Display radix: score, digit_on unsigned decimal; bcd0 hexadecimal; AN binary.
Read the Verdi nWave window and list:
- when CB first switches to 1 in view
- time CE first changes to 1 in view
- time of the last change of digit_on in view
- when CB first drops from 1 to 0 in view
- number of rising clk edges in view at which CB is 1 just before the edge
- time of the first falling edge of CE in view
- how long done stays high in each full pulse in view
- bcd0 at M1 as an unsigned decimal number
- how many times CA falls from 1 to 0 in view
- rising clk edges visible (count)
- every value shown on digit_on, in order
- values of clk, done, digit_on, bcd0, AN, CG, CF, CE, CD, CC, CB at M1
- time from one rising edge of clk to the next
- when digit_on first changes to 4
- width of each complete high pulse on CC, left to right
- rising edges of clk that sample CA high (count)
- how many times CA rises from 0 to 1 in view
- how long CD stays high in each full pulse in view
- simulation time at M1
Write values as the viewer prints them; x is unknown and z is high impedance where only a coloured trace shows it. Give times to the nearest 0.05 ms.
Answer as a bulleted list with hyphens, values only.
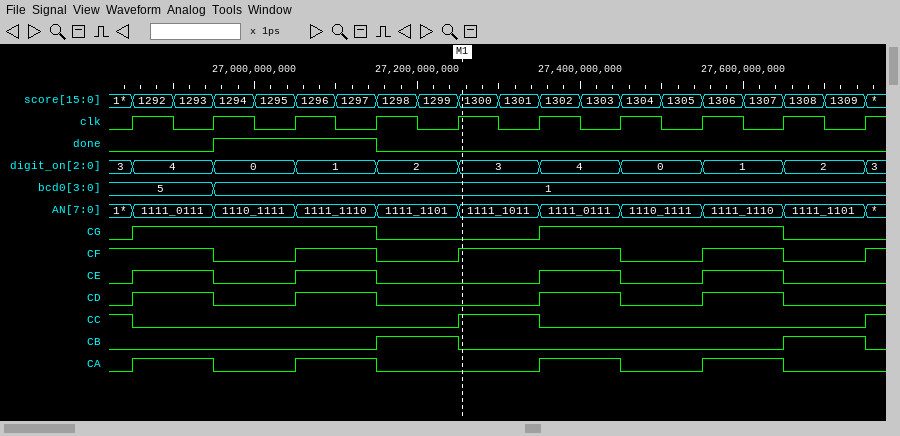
- 27.15 ms
- 26.85 ms
- 27.75 ms
- 27.25 ms
- 2
- 26.95 ms
- 0.2 ms
- 1
- 4
- 10
- 3, 4, 0, 1, 2, 3, 4, 0, 1, 2, 3
- clk=1, done=0, digit_on=3, bcd0=1, AN=1111_1011, CG=0, CF=1, CE=0, CD=0, CC=1, CB=0
- 0.1 ms
- 26.85 ms
- 0.1 ms
- 4
- 4
- 0.1 ms, 0.1 ms, 0.1 ms, 0.1 ms
- 27.25 ms
